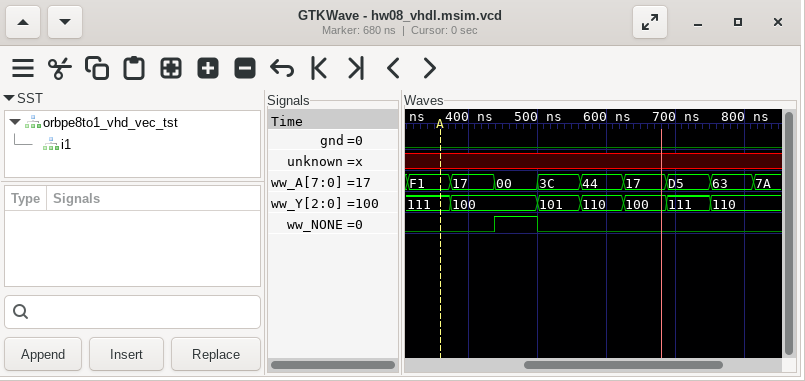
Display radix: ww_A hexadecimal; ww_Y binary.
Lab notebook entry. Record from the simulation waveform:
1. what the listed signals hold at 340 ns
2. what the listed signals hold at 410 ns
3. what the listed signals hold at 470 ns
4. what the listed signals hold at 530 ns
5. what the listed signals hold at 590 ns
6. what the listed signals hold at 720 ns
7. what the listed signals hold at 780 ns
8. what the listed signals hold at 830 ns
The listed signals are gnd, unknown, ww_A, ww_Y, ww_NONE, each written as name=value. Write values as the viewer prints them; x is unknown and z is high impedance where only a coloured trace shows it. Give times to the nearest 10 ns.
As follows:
gnd=0, unknown=x, ww_A=F1, ww_Y=111, ww_NONE=0
gnd=0, unknown=x, ww_A=17, ww_Y=100, ww_NONE=0
gnd=0, unknown=x, ww_A=00, ww_Y=100, ww_NONE=1
gnd=0, unknown=x, ww_A=3C, ww_Y=101, ww_NONE=0
gnd=0, unknown=x, ww_A=44, ww_Y=110, ww_NONE=0
gnd=0, unknown=x, ww_A=D5, ww_Y=111, ww_NONE=0
gnd=0, unknown=x, ww_A=63, ww_Y=110, ww_NONE=0
gnd=0, unknown=x, ww_A=7A, ww_Y=110, ww_NONE=0
